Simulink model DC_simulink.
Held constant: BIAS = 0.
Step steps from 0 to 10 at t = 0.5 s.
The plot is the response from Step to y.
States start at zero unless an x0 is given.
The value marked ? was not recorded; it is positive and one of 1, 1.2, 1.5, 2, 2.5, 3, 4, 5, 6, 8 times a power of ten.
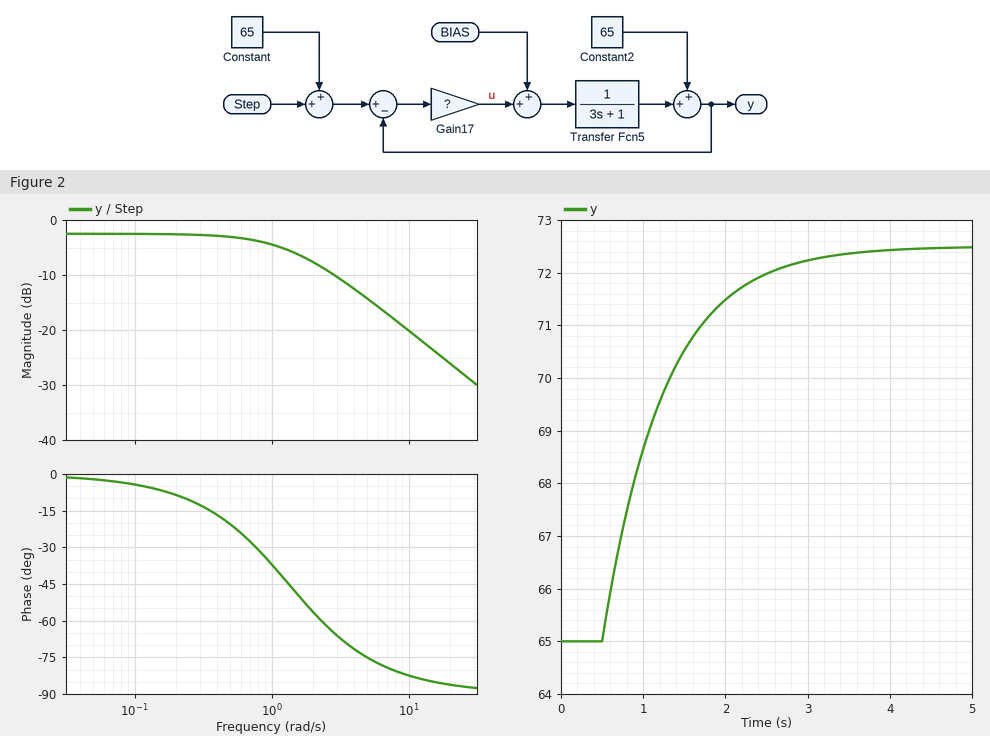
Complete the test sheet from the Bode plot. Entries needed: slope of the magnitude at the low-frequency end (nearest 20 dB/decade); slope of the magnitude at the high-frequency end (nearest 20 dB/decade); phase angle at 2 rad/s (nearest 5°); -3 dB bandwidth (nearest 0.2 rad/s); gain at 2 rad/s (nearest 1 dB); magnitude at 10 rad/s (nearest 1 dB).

0 dB/decade
-20 dB/decade
-55°
1.4 rad/s
-8 dB
-20 dB
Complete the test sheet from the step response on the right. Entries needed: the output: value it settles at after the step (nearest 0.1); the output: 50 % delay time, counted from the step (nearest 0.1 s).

72.5
0.5 s
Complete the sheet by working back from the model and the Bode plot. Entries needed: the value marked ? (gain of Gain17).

3
